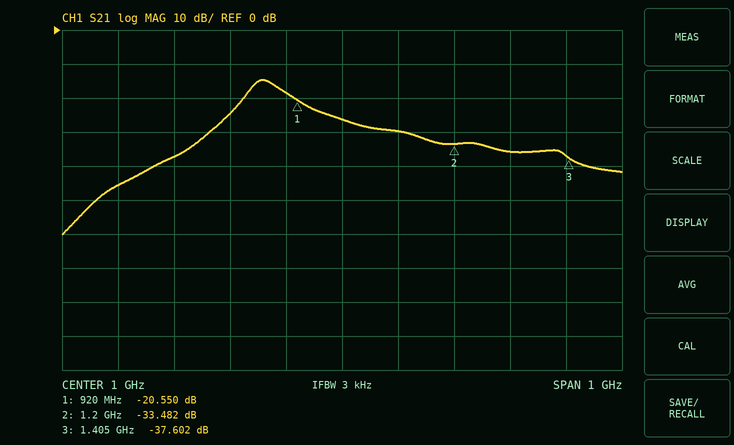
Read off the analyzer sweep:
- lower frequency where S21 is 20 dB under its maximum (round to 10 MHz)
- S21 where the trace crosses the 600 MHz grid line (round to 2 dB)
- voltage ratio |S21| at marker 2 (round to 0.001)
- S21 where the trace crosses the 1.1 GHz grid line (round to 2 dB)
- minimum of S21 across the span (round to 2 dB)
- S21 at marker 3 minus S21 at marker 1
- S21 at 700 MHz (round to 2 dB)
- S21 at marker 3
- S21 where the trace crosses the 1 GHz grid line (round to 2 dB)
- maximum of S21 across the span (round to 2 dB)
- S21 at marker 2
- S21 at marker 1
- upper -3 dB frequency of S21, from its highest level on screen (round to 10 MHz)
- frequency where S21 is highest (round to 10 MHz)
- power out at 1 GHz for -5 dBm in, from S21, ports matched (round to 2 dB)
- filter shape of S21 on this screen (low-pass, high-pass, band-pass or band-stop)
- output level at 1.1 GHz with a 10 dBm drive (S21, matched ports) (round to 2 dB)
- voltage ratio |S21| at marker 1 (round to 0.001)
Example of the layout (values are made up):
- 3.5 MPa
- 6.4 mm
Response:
- 730 MHz
- -46 dB
- 0.021
- -30 dB
- -60 dB
- -17.052 dB
- -38 dB
- -37.602 dB
- -26 dB
- -14 dB
- -33.482 dB
- -20.550 dB
- 890 MHz
- 860 MHz
- -32 dBm
- band-pass
- -20 dBm
- 0.094
